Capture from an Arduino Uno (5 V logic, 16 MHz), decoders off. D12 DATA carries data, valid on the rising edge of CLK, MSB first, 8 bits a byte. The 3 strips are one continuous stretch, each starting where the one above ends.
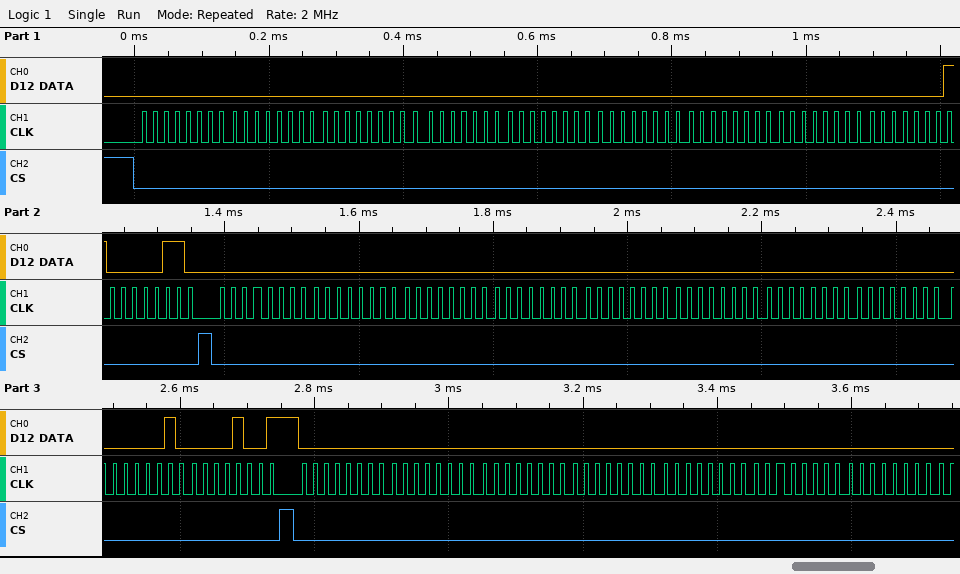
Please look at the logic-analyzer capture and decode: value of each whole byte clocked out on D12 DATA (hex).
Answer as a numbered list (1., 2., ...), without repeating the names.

1. 00 00 00 00 00 00 00 00 01 06 00 00 00 00 00 00 00 00 02 09 00 00 00 00 00 00 00
